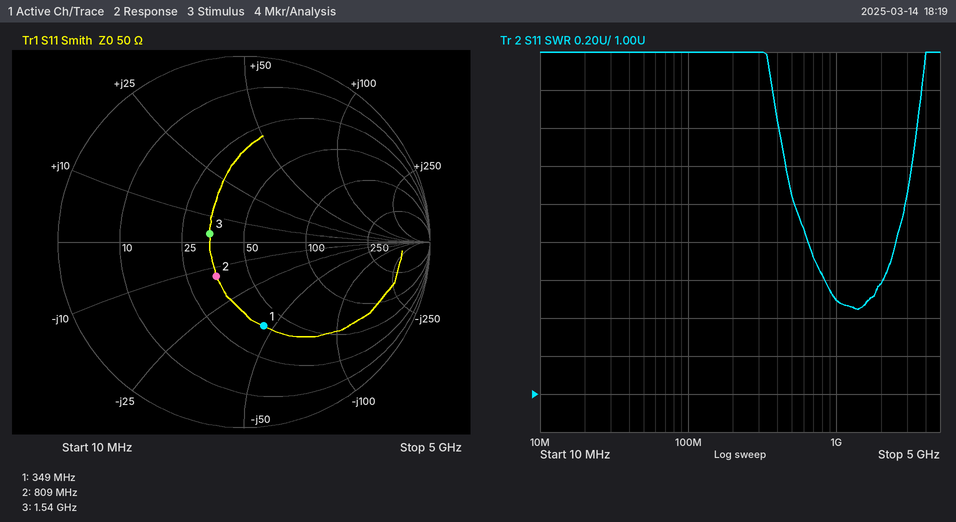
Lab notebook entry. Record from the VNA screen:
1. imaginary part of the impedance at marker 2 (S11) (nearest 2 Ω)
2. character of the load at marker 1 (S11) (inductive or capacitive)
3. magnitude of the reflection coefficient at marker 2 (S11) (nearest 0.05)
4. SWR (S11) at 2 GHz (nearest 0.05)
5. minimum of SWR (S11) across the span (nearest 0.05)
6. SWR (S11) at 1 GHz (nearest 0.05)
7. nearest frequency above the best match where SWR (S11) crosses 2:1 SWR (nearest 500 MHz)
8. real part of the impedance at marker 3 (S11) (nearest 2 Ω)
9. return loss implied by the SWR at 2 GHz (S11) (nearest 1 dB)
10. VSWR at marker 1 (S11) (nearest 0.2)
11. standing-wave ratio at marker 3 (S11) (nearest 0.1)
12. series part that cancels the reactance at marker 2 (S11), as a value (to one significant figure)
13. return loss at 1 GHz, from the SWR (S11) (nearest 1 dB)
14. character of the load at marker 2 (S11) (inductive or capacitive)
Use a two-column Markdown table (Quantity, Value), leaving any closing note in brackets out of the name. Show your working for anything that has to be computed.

| Quantity | Value |
|---|---|
| imaginary part of the impedance at marker 2 (S11) | -14 Ω |
| character of the load at marker 1 (S11) | capacitive |
| magnitude of the reflection coefficient at marker 2 (S11) | 0.25 |
| SWR (S11) at 2 GHz | 1.60 |
| minimum of SWR (S11) across the span | 1.45 |
| SWR (S11) at 1 GHz | 1.50 |
| nearest frequency above the best match where SWR (S11) crosses 2:1 SWR | 3.0 GHz |
| real part of the impedance at marker 3 (S11) | 34 Ω |
| return loss implied by the SWR at 2 GHz (S11) | −20 log10((1.6 − 1)/(1.6 + 1)) ≈ 13 dB |
| VSWR at marker 1 (S11) | 2.8 |
| standing-wave ratio at marker 3 (S11) | 1.5 |
| series part that cancels the reactance at marker 2 (S11), as a value | L = 14 Ω/(2π × 809 MHz) ≈ 3 nH |
| return loss at 1 GHz, from the SWR (S11) | −20 log10((1.5 − 1)/(1.5 + 1)) ≈ 14 dB |
| character of the load at marker 2 (S11) | capacitive |
